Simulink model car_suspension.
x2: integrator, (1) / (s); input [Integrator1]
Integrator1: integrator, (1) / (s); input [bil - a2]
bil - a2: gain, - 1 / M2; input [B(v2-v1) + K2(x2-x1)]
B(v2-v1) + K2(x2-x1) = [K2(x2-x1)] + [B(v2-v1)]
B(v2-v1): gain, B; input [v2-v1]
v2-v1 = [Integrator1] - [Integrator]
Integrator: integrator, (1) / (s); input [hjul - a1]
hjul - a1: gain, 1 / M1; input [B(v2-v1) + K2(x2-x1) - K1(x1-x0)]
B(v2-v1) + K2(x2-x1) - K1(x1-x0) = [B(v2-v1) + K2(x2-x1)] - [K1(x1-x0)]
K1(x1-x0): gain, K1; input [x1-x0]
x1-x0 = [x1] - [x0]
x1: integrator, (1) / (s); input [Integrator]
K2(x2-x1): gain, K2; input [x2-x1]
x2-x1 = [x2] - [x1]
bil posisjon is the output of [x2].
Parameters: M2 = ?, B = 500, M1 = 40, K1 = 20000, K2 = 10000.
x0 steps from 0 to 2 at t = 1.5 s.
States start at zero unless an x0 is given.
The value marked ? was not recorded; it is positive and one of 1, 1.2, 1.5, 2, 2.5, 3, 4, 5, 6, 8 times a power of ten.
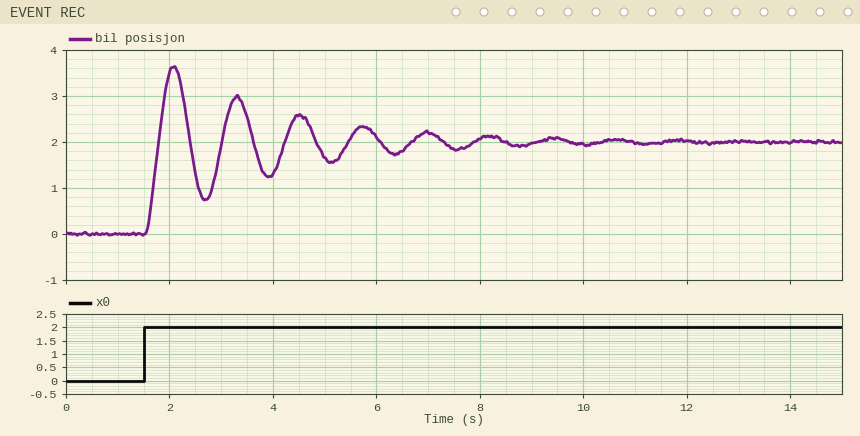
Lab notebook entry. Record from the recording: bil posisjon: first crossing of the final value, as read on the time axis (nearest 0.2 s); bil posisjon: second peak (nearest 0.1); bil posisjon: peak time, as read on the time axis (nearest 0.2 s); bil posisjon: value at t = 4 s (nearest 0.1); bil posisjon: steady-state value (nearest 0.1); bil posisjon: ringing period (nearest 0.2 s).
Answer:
1.8 s
3.0
2.0 s
1.3
2.0
1.2 s
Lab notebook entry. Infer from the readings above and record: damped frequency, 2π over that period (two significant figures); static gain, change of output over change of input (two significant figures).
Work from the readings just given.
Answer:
5.2 rad/s
1.0
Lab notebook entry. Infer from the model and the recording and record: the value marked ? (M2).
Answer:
250
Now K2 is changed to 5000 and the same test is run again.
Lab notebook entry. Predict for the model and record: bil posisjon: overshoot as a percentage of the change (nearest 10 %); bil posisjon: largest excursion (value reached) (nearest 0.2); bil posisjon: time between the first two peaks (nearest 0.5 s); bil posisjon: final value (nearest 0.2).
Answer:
70 %
3.4
1.5 s
2.0
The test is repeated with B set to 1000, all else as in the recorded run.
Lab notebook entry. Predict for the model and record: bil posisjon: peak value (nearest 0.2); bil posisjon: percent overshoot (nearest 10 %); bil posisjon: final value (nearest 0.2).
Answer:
3.4
70 %
2.0
